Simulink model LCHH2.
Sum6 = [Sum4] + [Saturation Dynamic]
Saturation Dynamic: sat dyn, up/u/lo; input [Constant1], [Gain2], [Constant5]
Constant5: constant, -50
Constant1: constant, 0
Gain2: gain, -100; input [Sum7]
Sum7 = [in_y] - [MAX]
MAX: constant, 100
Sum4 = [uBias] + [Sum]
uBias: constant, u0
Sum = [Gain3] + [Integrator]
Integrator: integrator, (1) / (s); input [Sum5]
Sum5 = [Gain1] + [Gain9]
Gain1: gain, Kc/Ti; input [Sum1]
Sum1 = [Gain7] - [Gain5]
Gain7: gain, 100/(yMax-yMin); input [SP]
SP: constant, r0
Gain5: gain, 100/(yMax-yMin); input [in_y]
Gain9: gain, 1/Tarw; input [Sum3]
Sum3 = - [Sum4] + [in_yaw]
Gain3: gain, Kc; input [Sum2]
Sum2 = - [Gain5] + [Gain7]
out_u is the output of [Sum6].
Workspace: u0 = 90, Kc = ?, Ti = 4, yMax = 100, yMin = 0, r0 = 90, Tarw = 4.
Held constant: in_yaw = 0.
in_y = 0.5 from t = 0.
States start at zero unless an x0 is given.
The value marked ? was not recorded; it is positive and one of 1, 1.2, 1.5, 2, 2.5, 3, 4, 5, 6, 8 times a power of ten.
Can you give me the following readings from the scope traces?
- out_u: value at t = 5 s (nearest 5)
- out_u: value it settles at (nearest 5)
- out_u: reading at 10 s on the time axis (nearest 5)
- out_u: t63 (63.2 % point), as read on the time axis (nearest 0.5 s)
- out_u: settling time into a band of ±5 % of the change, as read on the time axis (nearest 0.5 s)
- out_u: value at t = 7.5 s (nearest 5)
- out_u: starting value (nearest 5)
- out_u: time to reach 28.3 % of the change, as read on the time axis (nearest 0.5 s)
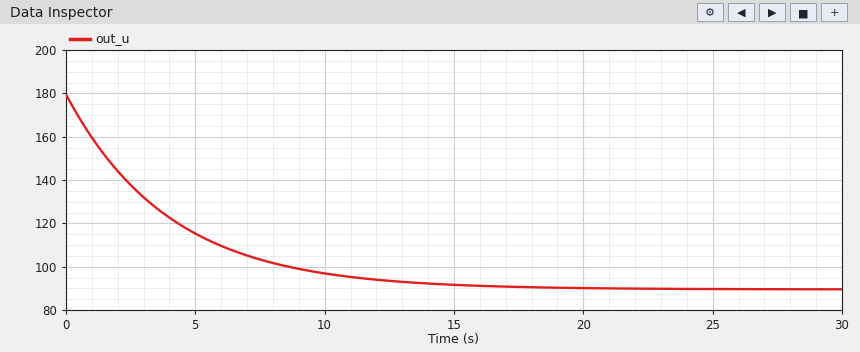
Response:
115
90
95
4.0 s
12.0 s
105
180
1.5 s
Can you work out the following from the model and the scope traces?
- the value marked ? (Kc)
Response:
1
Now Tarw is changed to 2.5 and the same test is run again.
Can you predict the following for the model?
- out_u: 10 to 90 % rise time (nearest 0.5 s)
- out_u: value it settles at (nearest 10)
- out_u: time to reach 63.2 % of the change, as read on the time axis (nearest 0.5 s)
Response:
5.5 s
60
2.5 s
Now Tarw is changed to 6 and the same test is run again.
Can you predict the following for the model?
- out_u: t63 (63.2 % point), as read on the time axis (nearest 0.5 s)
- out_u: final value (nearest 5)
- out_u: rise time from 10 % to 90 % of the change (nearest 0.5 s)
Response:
6.0 s
135
13.0 s
